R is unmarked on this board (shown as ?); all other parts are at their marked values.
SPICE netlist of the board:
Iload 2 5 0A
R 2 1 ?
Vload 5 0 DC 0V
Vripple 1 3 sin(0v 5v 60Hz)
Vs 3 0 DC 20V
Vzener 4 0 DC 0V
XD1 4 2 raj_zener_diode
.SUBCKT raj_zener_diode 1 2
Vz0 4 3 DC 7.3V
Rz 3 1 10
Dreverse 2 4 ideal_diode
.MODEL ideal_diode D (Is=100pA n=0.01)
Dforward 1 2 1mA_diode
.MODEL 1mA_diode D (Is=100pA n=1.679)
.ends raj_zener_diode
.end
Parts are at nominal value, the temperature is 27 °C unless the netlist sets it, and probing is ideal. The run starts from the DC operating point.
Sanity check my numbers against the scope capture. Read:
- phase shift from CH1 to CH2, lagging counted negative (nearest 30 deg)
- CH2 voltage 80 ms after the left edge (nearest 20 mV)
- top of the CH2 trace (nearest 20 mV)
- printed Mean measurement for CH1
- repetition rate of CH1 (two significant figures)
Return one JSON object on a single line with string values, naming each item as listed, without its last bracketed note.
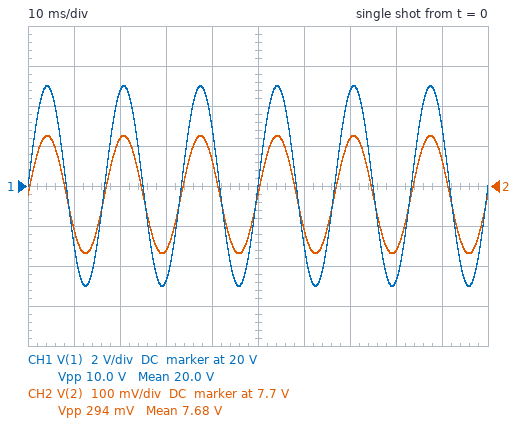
{"phase shift from CH1 to CH2, lagging counted negative": "0 deg", "CH2 voltage 80 ms after the left edge": "7.54 V", "top of the CH2 trace": "7.82 V", "printed Mean measurement for CH1": "20.0 V", "repetition rate of CH1": "60 Hz"}
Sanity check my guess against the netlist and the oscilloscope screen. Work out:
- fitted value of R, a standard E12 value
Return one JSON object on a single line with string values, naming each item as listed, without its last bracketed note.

{"fitted value of R, a standard E12 value": "330 Ω"}
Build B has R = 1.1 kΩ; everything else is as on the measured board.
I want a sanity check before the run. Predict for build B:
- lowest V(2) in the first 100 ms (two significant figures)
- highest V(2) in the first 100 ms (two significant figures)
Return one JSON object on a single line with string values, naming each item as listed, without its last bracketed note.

{"lowest V(2) in the first 100 ms": "7.4 V", "highest V(2) in the first 100 ms": "7.5 V"}
